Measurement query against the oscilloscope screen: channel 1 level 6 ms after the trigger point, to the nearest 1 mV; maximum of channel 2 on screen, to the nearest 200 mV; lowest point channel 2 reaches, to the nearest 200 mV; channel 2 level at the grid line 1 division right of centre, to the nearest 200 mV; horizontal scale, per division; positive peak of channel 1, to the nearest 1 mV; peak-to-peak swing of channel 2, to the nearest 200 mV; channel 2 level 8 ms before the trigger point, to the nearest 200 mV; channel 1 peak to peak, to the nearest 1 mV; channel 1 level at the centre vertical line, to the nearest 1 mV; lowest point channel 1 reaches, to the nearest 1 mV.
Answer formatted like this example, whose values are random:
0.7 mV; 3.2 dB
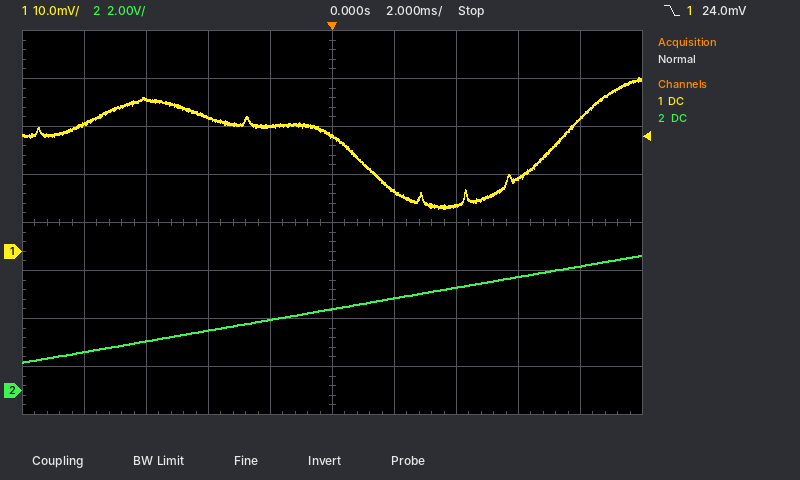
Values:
15 mV; 5.6 V; 1.2 V; 3.8 V; 2 ms; 36 mV; 4.4 V; 1.6 V; 27 mV; 24 mV; 9 mV
